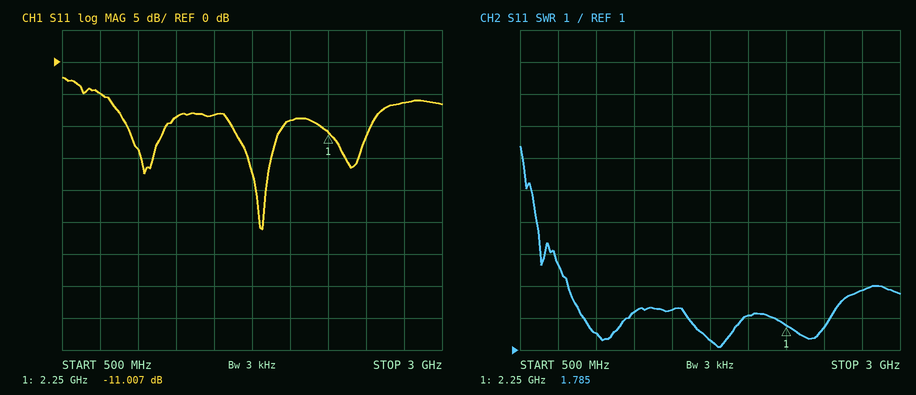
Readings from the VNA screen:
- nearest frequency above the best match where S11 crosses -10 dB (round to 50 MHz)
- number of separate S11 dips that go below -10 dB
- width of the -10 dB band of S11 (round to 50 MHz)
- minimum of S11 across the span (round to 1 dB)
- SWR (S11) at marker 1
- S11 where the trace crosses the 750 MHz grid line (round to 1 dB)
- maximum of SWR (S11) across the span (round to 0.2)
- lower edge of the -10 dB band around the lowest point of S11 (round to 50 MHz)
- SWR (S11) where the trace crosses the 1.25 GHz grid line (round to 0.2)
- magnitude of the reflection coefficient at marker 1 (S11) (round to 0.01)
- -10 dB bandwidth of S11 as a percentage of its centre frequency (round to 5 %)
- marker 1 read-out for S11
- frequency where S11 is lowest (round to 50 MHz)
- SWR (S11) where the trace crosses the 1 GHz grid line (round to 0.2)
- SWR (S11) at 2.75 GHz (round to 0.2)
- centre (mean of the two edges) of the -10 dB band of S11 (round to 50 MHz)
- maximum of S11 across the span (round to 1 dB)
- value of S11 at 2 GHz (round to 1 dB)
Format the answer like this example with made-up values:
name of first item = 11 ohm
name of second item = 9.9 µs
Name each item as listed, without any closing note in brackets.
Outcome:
nearest frequency above the best match where S11 crosses -10 dB = 1.95 GHz
number of separate S11 dips that go below -10 dB = 3
width of the -10 dB band of S11 = 350 MHz
minimum of S11 across the span = -26 dB
SWR (S11) at marker 1 = 1.785
S11 where the trace crosses the 750 MHz grid line = -5 dB
maximum of SWR (S11) across the span = 7.4
lower edge of the -10 dB band around the lowest point of S11 = 1.60 GHz
SWR (S11) where the trace crosses the 1.25 GHz grid line = 2.2
magnitude of the reflection coefficient at marker 1 (S11) = 0.28
-10 dB bandwidth of S11 as a percentage of its centre frequency = 20 %
marker 1 read-out for S11 = -11.007 dB
frequency where S11 is lowest = 1.80 GHz
SWR (S11) where the trace crosses the 1 GHz grid line = 1.6
SWR (S11) at 2.75 GHz = 2.8
centre (mean of the two edges) of the -10 dB band of S11 = 1.80 GHz
maximum of S11 across the span = -2 dB
value of S11 at 2 GHz = -9 dB
